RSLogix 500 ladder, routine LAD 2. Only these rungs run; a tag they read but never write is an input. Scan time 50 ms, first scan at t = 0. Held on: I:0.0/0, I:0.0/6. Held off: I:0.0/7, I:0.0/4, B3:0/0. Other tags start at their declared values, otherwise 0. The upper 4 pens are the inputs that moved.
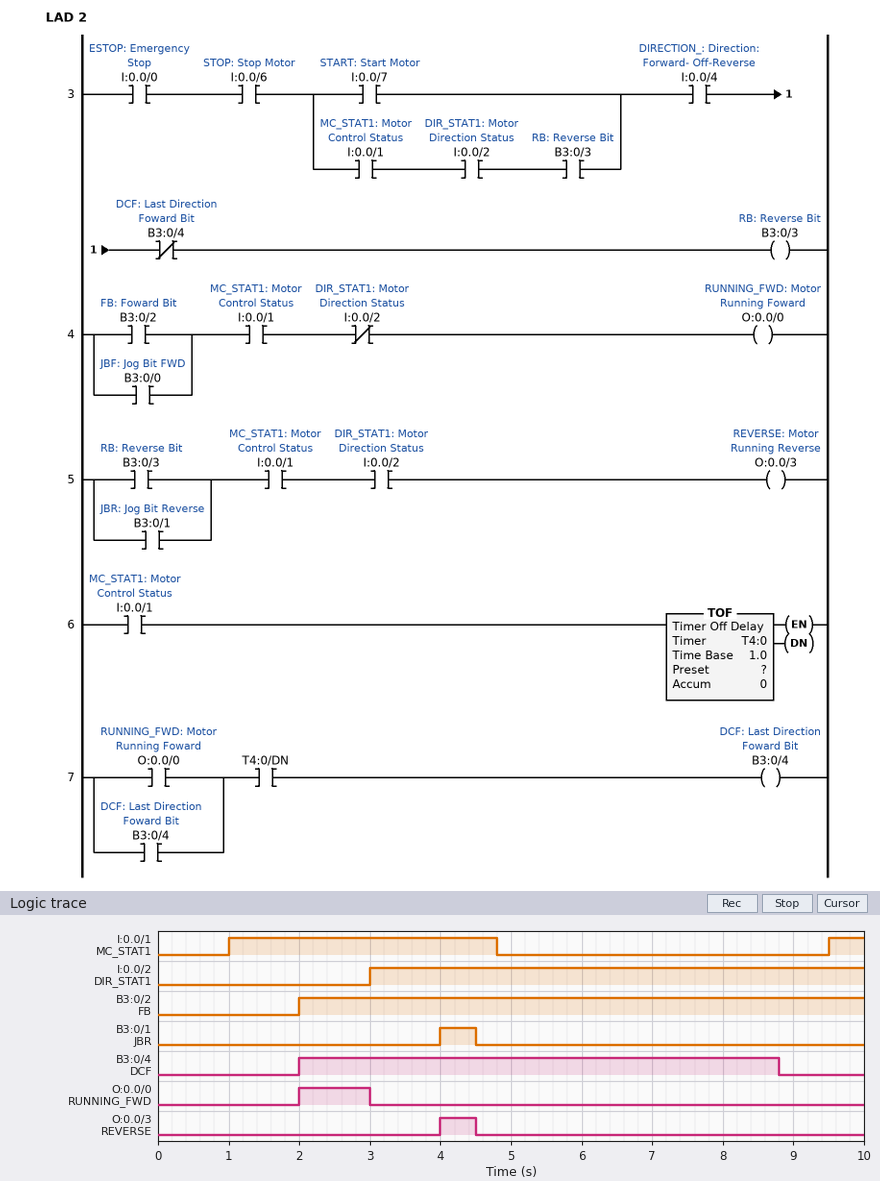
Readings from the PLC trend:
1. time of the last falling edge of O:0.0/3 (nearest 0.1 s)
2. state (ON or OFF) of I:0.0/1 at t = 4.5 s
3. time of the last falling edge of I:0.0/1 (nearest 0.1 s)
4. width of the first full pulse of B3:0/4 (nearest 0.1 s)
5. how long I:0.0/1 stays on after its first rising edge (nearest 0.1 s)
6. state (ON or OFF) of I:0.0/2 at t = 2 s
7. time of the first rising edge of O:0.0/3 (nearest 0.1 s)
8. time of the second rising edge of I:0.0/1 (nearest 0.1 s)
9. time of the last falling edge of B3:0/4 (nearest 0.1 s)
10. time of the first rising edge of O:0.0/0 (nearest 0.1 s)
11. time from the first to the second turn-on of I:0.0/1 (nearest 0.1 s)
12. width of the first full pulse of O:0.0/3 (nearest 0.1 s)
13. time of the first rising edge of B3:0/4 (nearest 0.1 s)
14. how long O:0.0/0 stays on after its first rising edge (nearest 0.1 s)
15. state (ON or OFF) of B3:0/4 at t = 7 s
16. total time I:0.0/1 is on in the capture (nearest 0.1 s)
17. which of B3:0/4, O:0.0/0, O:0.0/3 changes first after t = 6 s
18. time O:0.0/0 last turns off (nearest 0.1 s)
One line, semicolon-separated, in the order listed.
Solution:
4.5 s; ON; 4.8 s; 6.8 s; 3.8 s; OFF; 4.0 s; 9.5 s; 8.8 s; 2.0 s; 8.5 s; 0.5 s; 2.0 s; 1.0 s; ON; 4.3 s; B3:0/4; 3.0 s
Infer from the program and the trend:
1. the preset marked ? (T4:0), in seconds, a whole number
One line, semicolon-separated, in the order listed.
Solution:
4 s
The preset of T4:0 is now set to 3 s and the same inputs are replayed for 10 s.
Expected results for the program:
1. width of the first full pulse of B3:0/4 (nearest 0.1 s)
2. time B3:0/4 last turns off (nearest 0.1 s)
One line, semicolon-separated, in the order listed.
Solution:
5.8 s; 7.8 s
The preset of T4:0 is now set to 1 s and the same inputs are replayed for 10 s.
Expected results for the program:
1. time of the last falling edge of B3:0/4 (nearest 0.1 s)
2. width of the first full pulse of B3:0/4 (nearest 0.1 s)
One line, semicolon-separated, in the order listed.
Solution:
5.8 s; 3.8 s
